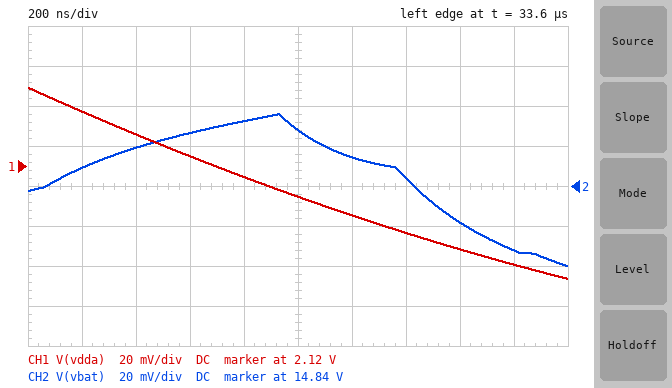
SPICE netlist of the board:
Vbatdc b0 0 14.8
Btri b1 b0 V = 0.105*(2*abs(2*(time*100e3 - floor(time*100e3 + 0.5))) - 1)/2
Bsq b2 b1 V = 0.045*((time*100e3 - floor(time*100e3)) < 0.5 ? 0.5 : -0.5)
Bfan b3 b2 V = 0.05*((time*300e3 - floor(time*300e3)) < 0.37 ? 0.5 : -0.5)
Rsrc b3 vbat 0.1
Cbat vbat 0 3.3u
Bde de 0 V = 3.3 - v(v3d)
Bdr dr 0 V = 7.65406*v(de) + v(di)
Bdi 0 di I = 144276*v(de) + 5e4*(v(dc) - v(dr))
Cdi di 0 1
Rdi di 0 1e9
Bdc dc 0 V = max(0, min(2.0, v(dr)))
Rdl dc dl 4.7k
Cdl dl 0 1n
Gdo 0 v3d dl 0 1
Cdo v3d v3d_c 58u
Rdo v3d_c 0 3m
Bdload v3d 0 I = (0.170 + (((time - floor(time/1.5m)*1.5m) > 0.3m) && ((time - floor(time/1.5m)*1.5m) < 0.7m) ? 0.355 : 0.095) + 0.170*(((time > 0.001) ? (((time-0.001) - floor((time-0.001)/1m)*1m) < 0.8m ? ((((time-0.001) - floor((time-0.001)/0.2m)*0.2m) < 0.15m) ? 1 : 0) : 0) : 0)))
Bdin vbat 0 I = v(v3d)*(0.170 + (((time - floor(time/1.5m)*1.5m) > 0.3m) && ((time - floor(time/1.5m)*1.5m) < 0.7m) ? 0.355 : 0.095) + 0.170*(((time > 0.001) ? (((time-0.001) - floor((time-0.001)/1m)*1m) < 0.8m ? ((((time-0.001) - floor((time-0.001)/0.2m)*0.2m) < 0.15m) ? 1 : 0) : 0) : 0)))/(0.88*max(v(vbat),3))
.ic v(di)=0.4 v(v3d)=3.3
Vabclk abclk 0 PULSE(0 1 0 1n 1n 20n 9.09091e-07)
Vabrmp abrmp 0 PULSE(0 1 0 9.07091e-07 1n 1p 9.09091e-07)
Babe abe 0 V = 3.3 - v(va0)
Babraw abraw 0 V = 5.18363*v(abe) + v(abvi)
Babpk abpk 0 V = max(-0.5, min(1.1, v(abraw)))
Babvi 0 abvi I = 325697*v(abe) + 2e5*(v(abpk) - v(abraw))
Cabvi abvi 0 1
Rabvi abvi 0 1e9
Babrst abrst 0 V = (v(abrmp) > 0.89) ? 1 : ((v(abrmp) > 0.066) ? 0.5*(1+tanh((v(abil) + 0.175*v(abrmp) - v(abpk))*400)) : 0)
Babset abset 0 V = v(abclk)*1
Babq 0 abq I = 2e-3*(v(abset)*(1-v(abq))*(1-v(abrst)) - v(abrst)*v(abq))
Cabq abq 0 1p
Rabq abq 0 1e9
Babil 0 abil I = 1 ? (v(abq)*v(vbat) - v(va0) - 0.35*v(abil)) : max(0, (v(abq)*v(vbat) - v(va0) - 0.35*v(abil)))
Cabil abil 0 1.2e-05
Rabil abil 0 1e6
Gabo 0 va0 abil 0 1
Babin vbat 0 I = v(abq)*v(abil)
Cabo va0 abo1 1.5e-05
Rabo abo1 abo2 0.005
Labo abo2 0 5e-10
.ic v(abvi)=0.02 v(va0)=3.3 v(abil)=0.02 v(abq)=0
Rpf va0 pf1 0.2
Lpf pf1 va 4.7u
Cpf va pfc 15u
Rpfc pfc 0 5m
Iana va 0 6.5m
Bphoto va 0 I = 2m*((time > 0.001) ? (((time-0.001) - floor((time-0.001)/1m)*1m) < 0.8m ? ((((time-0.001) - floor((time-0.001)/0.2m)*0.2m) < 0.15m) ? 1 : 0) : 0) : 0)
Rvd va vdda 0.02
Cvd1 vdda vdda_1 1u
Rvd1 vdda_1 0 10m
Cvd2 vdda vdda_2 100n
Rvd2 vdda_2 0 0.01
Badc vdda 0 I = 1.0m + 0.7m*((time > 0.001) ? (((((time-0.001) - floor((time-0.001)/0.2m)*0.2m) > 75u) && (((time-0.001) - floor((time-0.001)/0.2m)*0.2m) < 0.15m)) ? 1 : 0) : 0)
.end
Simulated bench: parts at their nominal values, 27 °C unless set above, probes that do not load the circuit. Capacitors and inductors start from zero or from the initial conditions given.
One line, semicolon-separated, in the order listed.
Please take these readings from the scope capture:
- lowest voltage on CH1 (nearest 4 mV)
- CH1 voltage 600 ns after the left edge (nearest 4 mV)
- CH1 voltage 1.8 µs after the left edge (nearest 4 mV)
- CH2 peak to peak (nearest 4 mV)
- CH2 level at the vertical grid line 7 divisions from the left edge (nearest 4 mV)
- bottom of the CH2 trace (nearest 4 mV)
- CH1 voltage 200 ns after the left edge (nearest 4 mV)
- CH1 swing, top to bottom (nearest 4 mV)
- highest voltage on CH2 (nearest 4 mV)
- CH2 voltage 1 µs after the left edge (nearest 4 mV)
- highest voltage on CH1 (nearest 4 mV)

2.064 V; 2.124 V; 2.072 V; 76 mV; 14.844 V; 14.800 V; 2.148 V; 96 mV; 14.876 V; 14.868 V; 2.160 V
